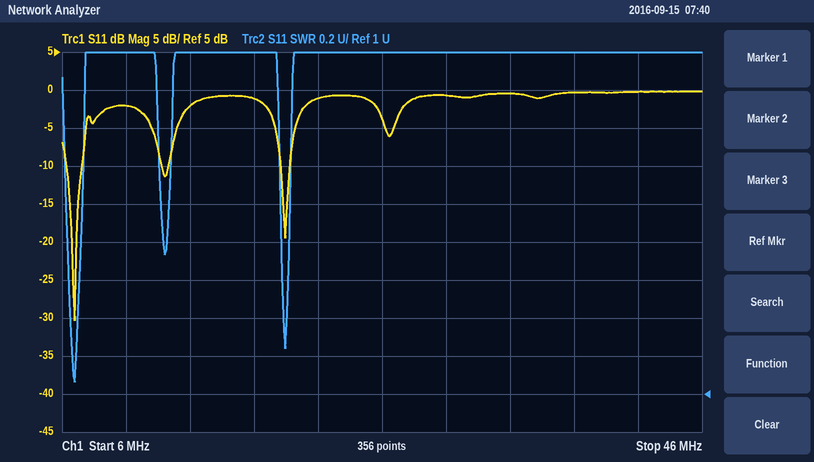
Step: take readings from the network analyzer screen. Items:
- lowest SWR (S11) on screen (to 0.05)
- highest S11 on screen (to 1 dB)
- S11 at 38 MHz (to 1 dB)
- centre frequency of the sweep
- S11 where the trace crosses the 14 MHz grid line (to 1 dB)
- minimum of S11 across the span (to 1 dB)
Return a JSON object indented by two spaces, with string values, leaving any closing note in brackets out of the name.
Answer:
{
  "lowest SWR (S11) on screen": "1.05",
  "highest S11 on screen": "0 dB",
  "S11 at 38 MHz": "0 dB",
  "centre frequency of the sweep": "26 MHz",
  "S11 where the trace crosses the 14 MHz grid line": "-2 dB",
  "minimum of S11 across the span": "-30 dB"
}
